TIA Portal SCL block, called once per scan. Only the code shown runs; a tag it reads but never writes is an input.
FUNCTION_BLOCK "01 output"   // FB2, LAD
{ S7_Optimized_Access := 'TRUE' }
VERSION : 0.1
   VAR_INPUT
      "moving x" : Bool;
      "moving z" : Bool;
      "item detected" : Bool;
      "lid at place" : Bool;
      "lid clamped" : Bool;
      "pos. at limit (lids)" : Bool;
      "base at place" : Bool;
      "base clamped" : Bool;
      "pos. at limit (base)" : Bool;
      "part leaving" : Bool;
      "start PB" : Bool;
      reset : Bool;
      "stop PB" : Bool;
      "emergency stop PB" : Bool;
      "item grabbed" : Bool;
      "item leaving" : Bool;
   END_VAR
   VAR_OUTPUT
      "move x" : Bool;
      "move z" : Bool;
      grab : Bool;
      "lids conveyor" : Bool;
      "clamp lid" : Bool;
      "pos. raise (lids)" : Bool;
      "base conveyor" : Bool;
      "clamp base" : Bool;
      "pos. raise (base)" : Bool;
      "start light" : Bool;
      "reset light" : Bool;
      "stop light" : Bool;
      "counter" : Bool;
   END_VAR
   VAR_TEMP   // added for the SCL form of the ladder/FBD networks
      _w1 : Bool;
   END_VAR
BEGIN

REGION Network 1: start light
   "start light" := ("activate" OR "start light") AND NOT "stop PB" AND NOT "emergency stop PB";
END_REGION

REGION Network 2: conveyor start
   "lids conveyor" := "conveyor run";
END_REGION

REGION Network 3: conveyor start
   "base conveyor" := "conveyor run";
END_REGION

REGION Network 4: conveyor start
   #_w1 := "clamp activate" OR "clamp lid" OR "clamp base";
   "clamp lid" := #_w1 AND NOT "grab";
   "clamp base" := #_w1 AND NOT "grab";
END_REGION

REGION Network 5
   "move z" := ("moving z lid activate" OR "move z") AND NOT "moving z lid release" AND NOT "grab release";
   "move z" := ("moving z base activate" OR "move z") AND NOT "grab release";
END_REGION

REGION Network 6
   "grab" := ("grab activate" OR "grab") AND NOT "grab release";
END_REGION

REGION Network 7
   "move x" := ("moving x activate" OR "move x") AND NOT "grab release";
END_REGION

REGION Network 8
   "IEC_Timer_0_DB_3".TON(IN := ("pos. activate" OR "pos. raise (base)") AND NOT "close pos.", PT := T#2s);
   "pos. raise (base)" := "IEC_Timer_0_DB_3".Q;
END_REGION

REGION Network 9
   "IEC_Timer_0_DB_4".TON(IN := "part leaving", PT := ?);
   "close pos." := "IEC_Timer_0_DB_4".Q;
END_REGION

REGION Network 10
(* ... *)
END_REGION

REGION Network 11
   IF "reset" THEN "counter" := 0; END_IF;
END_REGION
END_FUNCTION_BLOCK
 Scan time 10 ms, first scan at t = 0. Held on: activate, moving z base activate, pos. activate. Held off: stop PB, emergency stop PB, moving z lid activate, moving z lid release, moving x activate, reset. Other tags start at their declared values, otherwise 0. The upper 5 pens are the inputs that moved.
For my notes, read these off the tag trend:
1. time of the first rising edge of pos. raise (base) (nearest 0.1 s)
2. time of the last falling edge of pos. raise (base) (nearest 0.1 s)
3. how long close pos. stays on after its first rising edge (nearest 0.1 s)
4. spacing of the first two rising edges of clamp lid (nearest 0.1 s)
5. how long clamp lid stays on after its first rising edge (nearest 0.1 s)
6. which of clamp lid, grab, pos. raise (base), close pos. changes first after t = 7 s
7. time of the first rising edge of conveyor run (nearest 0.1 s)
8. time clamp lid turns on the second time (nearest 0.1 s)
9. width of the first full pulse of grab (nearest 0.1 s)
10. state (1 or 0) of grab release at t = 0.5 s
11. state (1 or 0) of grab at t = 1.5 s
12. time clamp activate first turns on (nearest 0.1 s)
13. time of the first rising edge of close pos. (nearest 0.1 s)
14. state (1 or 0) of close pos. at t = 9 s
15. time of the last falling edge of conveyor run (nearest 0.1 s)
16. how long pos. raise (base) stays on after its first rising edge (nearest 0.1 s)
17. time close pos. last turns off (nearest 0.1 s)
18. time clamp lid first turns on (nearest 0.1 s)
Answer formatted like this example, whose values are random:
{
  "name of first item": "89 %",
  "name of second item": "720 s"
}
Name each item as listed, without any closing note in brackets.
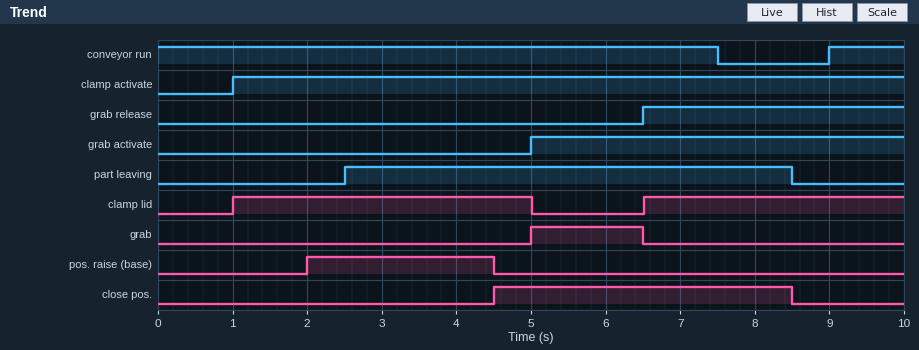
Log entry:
{
  "time of the first rising edge of pos. raise (base)": "2.0 s",
  "time of the last falling edge of pos. raise (base)": "4.5 s",
  "how long close pos. stays on after its first rising edge": "4.0 s",
  "spacing of the first two rising edges of clamp lid": "5.5 s",
  "how long clamp lid stays on after its first rising edge": "4.0 s",
  "which of clamp lid, grab, pos. raise (base), close pos. changes first after t = 7 s": "close pos.",
  "time of the first rising edge of conveyor run": "9.0 s",
  "time clamp lid turns on the second time": "6.5 s",
  "width of the first full pulse of grab": "1.5 s",
  "state (1 or 0) of grab release at t = 0.5 s": "0",
  "state (1 or 0) of grab at t = 1.5 s": "0",
  "time clamp activate first turns on": "1.0 s",
  "time of the first rising edge of close pos.": "4.5 s",
  "state (1 or 0) of close pos. at t = 9 s": "0",
  "time of the last falling edge of conveyor run": "7.5 s",
  "how long pos. raise (base) stays on after its first rising edge": "2.5 s",
  "time close pos. last turns off": "8.5 s",
  "time clamp lid first turns on": "1.0 s"
}
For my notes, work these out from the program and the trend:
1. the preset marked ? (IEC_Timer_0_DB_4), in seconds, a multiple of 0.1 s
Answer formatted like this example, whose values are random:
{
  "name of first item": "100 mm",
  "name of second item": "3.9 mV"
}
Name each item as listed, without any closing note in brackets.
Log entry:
{
  "the preset marked ? (IEC_Timer_0_DB_4), in seconds, a multiple of 0.1 s": "2.0 s"
}
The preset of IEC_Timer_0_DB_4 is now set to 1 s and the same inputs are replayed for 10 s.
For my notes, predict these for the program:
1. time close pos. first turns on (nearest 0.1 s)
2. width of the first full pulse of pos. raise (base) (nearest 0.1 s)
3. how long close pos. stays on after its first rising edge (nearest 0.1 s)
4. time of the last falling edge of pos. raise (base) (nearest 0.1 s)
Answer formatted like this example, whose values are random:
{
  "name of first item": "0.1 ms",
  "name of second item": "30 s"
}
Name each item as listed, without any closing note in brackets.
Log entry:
{
  "time close pos. first turns on": "3.5 s",
  "width of the first full pulse of pos. raise (base)": "1.5 s",
  "how long close pos. stays on after its first rising edge": "5.0 s",
  "time of the last falling edge of pos. raise (base)": "3.5 s"
}
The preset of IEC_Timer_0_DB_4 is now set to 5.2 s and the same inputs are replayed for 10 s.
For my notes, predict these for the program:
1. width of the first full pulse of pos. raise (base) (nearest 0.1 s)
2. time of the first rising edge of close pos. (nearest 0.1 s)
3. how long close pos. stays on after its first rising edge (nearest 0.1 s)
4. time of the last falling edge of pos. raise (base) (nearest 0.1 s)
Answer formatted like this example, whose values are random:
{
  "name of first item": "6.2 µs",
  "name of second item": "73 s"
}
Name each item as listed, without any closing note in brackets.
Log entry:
{
  "width of the first full pulse of pos. raise (base)": "5.7 s",
  "time of the first rising edge of close pos.": "7.7 s",
  "how long close pos. stays on after its first rising edge": "0.8 s",
  "time of the last falling edge of pos. raise (base)": "7.7 s"
}
